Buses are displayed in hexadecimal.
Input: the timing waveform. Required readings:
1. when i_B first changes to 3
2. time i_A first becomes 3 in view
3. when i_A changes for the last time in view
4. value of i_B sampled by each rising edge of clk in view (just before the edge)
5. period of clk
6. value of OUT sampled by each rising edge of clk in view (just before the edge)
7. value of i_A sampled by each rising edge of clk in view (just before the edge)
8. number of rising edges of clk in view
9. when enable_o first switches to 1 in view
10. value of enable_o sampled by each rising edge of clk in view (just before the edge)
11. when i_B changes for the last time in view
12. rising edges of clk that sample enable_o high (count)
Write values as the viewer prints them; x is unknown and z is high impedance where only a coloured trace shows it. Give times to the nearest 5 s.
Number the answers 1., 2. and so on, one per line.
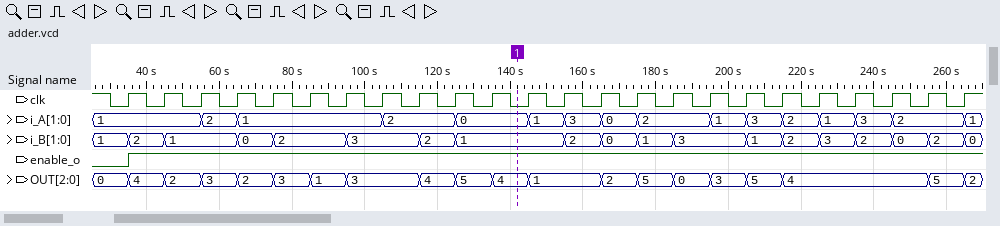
1. 95 s
2. 155 s
3. 265 s
4. 1, 2, 1, 1, 0, 2, 2, 3, 3, 2, 1, 1, 1, 2, 0, 1, 3, 3, 1, 2, 3, 2, 0, 2
5. 10 s
6. 0, 4, 2, 3, 2, 3, 1, 3, 3, 4, 5, 4, 1, 1, 2, 5, 0, 3, 5, 4, 4, 4, 4, 5
7. 1, 1, 1, 2, 1, 1, 1, 1, 2, 2, 0, 0, 1, 3, 0, 2, 2, 1, 3, 2, 1, 3, 2, 2
8. 24
9. 35 s
10. 0 1 1 1 1 1 1 1 1 1 1 1 1 1 1 1 1 1 1 1 1 1 1 1
11. 265 s
12. 23
